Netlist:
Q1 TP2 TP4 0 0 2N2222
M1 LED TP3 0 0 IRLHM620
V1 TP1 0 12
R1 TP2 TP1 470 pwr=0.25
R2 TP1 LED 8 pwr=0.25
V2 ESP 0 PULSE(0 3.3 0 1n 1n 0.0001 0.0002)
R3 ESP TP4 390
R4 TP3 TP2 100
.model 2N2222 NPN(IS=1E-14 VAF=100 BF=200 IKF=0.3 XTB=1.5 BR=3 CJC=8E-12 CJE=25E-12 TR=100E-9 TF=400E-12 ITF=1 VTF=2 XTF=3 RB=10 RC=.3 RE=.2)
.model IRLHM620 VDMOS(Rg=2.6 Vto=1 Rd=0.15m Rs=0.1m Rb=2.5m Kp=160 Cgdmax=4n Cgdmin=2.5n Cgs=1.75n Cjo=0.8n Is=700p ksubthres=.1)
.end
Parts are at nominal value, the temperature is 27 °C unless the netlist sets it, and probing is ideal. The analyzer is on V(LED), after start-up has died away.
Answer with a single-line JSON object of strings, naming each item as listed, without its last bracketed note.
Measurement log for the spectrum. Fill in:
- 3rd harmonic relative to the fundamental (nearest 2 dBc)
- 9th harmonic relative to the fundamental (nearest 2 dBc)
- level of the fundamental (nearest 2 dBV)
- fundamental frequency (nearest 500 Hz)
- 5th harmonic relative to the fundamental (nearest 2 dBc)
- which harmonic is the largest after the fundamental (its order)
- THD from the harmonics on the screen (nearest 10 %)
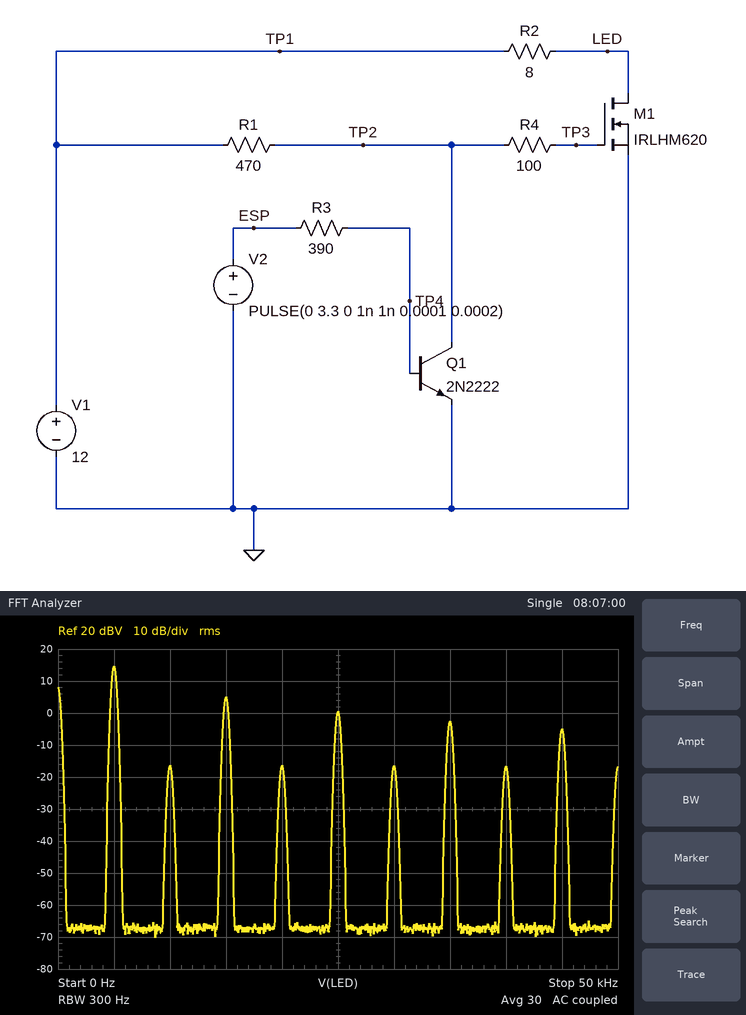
{"3rd harmonic relative to the fundamental": "-10 dBc", "9th harmonic relative to the fundamental": "-20 dBc", "level of the fundamental": "14 dBV", "fundamental frequency": "5.0 kHz", "5th harmonic relative to the fundamental": "-14 dBc", "which harmonic is the largest after the fundamental": "3", "THD from the harmonics on the screen": "40 %"}
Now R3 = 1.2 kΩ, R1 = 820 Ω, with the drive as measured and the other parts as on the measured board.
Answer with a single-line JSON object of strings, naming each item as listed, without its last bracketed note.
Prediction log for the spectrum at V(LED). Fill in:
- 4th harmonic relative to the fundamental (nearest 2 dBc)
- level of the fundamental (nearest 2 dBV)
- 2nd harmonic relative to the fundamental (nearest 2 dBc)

{"4th harmonic relative to the fundamental": "-34 dBc", "level of the fundamental": "14 dBV", "2nd harmonic relative to the fundamental": "-34 dBc"}
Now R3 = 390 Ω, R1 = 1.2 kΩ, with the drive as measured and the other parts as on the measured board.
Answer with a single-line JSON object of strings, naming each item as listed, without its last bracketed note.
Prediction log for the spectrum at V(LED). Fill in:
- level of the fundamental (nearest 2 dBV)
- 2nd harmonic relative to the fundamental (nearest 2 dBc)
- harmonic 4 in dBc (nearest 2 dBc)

{"level of the fundamental": "14 dBV", "2nd harmonic relative to the fundamental": "-44 dBc", "harmonic 4 in dBc": "-44 dBc"}
